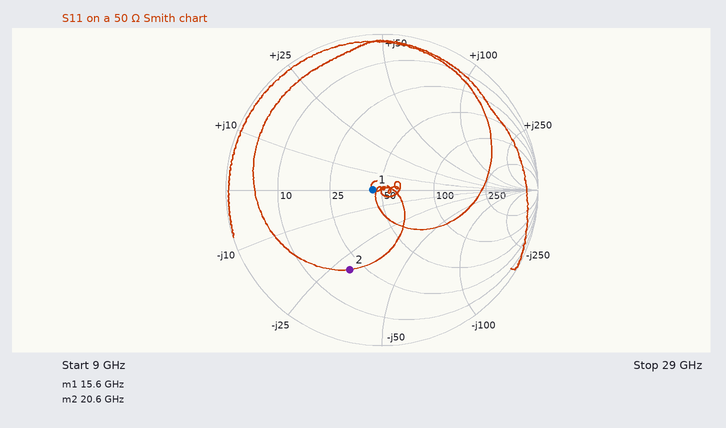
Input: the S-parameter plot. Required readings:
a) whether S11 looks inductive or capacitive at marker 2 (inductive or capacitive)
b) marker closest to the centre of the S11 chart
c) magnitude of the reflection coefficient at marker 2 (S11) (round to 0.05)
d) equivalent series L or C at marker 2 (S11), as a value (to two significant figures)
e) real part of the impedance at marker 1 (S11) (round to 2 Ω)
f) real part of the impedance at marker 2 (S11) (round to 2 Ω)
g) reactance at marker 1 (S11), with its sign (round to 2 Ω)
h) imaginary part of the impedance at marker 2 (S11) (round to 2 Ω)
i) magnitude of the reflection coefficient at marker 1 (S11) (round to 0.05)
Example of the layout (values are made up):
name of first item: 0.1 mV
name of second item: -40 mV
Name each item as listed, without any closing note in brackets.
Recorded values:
whether S11 looks inductive or capacitive at marker 2: capacitive
marker closest to the centre of the S11 chart: marker 1
magnitude of the reflection coefficient at marker 2 (S11): 0.55
equivalent series L or C at marker 2 (S11), as a value: 260 fF
real part of the impedance at marker 1 (S11): 44 Ω
real part of the impedance at marker 2 (S11): 20 Ω
reactance at marker 1 (S11), with its sign: 0 Ω
imaginary part of the impedance at marker 2 (S11): -30 Ω
magnitude of the reflection coefficient at marker 1 (S11): 0.05
